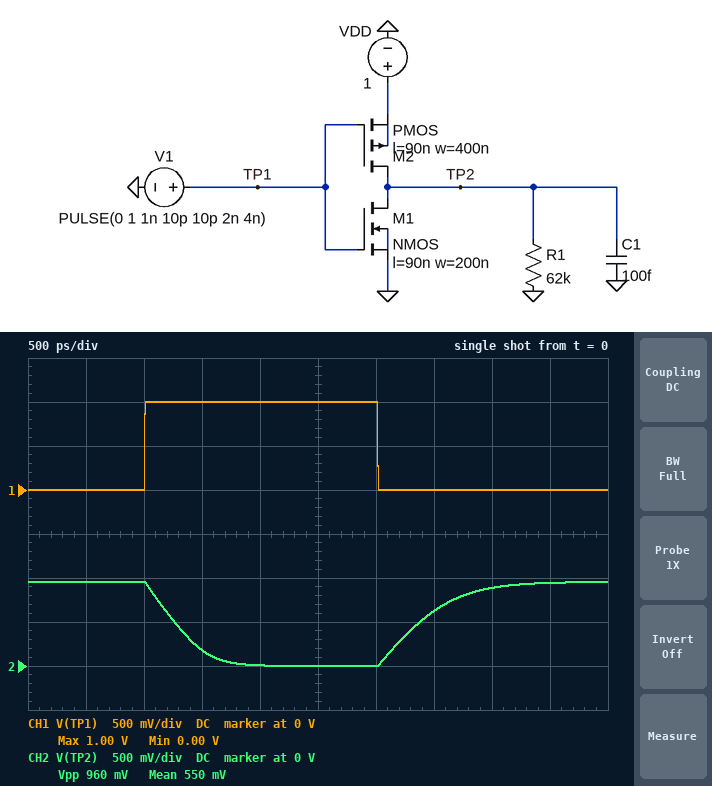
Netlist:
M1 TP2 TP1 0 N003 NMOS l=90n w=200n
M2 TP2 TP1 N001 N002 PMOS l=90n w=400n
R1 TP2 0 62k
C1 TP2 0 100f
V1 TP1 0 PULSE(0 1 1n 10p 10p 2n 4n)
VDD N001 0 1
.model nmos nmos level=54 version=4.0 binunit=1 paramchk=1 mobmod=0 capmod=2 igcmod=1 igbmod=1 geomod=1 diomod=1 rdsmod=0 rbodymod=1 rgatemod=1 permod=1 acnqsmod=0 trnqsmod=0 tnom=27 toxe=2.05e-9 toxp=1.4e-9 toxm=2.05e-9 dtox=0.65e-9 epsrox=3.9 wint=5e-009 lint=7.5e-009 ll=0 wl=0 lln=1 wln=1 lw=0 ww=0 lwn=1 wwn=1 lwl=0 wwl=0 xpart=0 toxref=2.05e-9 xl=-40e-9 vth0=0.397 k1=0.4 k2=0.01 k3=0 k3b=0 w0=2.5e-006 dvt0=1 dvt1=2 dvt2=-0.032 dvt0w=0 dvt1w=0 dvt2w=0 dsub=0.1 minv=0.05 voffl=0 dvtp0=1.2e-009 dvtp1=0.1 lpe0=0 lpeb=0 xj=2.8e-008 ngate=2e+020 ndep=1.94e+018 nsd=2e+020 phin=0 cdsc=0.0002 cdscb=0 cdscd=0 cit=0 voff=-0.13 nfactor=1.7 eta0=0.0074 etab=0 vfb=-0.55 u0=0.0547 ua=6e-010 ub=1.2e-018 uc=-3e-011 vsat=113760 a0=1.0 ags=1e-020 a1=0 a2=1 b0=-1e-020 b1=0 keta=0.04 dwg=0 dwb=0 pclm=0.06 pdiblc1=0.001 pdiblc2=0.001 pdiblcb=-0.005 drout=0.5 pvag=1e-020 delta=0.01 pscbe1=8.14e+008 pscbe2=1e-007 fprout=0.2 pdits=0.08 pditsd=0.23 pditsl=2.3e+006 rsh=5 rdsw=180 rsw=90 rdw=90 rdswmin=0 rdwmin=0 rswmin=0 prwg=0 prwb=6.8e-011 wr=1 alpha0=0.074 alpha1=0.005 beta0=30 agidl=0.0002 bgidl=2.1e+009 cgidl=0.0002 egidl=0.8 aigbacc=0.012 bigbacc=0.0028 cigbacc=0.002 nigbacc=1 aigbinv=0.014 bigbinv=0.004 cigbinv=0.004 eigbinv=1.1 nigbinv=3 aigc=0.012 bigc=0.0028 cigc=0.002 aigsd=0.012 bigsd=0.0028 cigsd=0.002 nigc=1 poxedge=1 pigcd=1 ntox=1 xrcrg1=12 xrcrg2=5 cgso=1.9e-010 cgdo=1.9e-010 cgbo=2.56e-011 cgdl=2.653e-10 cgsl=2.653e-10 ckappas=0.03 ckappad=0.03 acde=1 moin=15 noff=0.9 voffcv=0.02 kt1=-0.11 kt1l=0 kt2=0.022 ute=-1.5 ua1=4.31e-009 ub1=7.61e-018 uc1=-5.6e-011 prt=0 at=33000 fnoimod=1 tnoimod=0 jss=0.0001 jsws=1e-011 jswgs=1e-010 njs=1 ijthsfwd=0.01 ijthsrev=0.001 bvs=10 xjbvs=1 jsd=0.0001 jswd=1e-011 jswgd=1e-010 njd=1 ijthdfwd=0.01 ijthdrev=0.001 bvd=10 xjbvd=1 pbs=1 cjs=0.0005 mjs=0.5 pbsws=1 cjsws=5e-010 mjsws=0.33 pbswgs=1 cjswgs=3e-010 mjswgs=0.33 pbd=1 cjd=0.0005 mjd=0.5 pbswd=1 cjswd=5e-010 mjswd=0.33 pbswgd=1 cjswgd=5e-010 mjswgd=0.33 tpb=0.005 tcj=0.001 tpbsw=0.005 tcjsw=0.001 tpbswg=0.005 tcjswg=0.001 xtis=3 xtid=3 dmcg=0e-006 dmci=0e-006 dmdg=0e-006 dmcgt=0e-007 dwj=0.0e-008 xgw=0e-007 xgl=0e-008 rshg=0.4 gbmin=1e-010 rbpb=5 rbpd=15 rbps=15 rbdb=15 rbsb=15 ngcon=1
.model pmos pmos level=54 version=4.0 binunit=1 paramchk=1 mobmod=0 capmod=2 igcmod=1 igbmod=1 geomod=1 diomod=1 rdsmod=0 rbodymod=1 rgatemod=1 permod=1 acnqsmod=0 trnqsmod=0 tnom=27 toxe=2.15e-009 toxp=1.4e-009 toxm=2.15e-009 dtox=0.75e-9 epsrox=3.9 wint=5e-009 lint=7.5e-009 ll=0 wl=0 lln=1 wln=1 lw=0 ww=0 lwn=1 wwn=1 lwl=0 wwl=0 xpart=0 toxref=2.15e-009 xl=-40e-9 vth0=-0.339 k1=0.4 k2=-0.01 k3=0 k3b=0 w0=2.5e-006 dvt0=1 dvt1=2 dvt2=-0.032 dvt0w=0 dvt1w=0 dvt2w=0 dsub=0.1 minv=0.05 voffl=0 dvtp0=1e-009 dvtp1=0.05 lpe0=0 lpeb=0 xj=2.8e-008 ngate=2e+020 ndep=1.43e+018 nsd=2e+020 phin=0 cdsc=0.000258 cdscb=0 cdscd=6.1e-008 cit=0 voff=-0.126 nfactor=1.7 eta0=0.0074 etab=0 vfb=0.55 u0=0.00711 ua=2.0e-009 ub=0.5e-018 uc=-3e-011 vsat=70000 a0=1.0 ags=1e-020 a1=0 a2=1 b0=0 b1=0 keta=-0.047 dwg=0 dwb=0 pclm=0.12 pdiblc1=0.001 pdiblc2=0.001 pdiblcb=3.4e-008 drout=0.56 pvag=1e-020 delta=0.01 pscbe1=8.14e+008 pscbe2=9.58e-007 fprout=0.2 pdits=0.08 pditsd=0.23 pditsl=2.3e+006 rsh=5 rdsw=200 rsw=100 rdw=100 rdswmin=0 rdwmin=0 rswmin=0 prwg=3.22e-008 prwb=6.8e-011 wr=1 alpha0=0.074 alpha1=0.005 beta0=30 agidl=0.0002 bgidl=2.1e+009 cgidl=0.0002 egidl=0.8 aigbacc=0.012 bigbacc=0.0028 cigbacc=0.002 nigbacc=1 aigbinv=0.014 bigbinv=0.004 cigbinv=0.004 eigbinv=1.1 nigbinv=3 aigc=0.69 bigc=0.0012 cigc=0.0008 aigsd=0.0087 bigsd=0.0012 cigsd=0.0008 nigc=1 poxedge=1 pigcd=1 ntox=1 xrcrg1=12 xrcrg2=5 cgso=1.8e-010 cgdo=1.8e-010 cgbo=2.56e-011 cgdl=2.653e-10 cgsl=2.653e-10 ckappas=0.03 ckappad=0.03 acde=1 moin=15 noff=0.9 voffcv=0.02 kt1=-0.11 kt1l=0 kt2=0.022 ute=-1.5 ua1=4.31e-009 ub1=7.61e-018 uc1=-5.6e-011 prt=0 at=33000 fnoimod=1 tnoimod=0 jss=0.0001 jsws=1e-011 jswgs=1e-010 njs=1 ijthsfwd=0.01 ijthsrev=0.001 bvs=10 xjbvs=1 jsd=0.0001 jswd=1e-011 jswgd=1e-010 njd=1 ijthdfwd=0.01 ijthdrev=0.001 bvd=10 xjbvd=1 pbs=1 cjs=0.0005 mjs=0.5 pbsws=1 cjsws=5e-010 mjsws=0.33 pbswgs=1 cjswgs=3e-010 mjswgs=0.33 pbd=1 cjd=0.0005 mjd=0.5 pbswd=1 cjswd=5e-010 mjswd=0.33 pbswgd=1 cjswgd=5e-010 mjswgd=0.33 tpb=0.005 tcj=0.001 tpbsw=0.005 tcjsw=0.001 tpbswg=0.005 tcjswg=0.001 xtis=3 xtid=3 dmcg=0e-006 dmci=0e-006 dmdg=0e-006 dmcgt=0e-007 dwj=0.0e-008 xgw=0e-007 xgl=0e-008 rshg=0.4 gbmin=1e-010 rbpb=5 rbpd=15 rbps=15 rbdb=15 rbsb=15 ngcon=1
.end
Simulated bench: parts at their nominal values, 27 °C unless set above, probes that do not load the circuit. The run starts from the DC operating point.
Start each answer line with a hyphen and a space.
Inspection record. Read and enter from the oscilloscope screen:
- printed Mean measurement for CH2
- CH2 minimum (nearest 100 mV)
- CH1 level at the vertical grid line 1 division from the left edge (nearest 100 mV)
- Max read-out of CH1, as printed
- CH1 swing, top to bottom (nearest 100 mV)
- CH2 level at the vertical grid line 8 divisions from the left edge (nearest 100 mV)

- 550 mV
- 0 V
- 0 V
- 1.00 V
- 1.0 V
- 900 mV
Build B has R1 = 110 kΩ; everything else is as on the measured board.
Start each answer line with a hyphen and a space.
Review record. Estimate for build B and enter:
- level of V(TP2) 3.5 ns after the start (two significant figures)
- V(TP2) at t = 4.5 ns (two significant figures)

- 630 mV
- 960 mV
